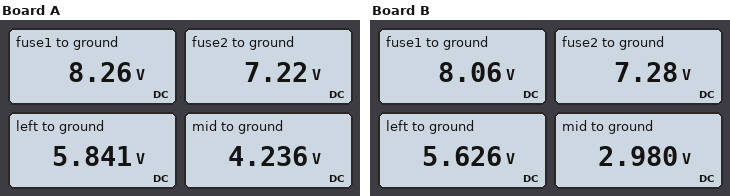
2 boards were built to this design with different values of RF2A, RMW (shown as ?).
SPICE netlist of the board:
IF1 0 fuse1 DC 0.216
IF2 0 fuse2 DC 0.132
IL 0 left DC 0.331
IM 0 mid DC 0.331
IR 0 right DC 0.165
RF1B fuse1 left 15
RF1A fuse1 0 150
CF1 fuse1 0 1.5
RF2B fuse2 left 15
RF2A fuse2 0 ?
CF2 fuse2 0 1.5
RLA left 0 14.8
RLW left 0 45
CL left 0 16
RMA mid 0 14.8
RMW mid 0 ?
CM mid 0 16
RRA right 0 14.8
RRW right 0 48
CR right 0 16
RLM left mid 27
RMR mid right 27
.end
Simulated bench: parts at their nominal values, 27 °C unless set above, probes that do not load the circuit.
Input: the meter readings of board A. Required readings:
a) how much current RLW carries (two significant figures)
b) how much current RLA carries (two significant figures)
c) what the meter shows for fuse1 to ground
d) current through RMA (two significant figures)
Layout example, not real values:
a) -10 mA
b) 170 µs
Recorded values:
a) 130 mA
b) 390 mA
c) 8.26 V
d) 290 mA
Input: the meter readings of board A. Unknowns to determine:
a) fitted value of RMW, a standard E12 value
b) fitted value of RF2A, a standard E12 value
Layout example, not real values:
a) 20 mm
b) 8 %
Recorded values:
a) 100 Ω
b) 180 Ω
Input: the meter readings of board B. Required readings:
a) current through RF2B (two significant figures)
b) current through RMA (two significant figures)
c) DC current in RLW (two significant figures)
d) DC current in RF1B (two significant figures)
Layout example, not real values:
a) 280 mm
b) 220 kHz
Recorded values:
a) 110 mA
b) 200 mA
c) 130 mA
d) 160 mA
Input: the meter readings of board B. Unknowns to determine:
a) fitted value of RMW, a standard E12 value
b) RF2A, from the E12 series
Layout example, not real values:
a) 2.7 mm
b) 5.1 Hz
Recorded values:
a) 15 Ω
b) 330 Ω
